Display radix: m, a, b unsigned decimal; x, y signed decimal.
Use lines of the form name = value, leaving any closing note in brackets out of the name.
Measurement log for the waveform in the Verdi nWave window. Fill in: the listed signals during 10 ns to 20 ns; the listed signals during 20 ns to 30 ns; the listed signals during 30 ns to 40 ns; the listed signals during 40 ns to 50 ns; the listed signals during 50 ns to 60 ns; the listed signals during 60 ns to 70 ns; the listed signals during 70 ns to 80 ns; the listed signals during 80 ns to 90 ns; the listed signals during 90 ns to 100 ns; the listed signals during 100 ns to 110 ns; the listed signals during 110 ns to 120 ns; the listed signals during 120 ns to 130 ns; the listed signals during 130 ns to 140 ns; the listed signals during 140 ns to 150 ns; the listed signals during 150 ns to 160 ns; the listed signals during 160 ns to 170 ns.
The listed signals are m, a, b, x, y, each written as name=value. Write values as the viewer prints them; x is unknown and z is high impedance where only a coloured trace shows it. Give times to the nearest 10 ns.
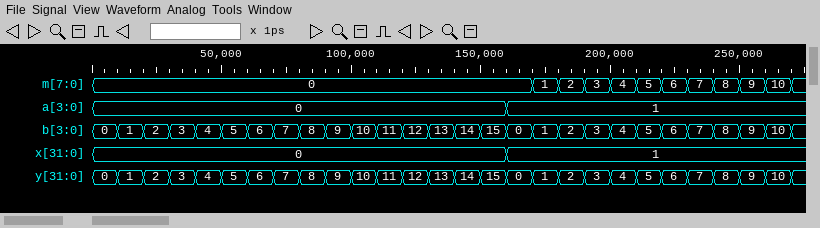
the listed signals during 10 ns to 20 ns = m=0, a=0, b=1, x=0, y=1
the listed signals during 20 ns to 30 ns = m=0, a=0, b=2, x=0, y=2
the listed signals during 30 ns to 40 ns = m=0, a=0, b=3, x=0, y=3
the listed signals during 40 ns to 50 ns = m=0, a=0, b=4, x=0, y=4
the listed signals during 50 ns to 60 ns = m=0, a=0, b=5, x=0, y=5
the listed signals during 60 ns to 70 ns = m=0, a=0, b=6, x=0, y=6
the listed signals during 70 ns to 80 ns = m=0, a=0, b=7, x=0, y=7
the listed signals during 80 ns to 90 ns = m=0, a=0, b=8, x=0, y=8
the listed signals during 90 ns to 100 ns = m=0, a=0, b=9, x=0, y=9
the listed signals during 100 ns to 110 ns = m=0, a=0, b=10, x=0, y=10
the listed signals during 110 ns to 120 ns = m=0, a=0, b=11, x=0, y=11
the listed signals during 120 ns to 130 ns = m=0, a=0, b=12, x=0, y=12
the listed signals during 130 ns to 140 ns = m=0, a=0, b=13, x=0, y=13
the listed signals during 140 ns to 150 ns = m=0, a=0, b=14, x=0, y=14
the listed signals during 150 ns to 160 ns = m=0, a=0, b=15, x=0, y=15
the listed signals during 160 ns to 170 ns = m=0, a=1, b=0, x=1, y=0
